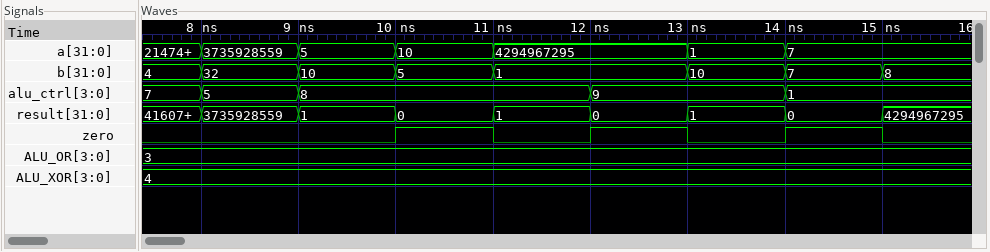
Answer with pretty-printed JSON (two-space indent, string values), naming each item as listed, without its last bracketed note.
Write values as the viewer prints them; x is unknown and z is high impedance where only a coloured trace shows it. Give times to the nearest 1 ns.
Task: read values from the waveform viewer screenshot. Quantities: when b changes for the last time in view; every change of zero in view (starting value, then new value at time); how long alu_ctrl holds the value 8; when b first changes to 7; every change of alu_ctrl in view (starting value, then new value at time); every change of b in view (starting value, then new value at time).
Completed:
{
  "when b changes for the last time in view": "15 ns",
  "every change of zero in view": "0, 1 at 10 ns, 0 at 11 ns, 1 at 12 ns, 0 at 13 ns, 1 at 14 ns, 0 at 15 ns",
  "how long alu_ctrl holds the value 8": "3 ns",
  "when b first changes to 7": "14 ns",
  "every change of alu_ctrl in view": "7, 5 at 8 ns, 8 at 9 ns, 9 at 12 ns, 1 at 14 ns",
  "every change of b in view": "4, 32 at 8 ns, 10 at 9 ns, 5 at 10 ns, 1 at 11 ns, 10 at 13 ns, 7 at 14 ns, 8 at 15 ns"
}
